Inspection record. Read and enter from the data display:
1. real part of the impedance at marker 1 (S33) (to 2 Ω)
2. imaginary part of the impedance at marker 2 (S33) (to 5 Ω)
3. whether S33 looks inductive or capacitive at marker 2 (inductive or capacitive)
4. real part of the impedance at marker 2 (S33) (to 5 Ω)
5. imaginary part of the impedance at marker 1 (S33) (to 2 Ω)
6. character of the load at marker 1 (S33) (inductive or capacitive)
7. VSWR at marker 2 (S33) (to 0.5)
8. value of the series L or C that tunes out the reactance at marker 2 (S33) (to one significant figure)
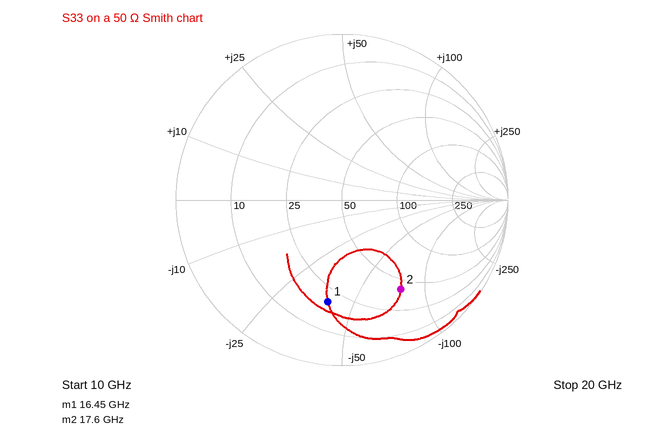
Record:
20 Ω
-75 Ω
capacitive
40 Ω
-40 Ω
capacitive
4.5
700 pH
